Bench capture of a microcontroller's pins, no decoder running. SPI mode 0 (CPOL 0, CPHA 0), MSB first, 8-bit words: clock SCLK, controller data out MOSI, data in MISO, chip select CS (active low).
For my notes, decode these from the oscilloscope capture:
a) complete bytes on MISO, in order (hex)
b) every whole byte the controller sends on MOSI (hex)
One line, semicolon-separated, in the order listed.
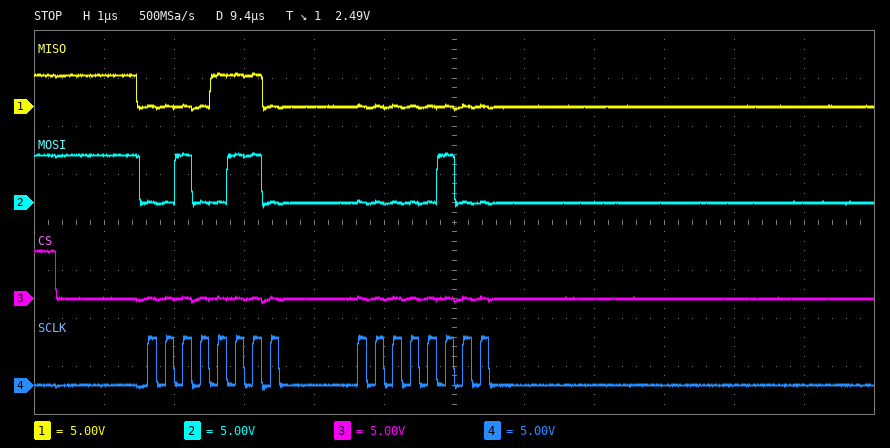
0x0E 0x00; 0x26 0x04
